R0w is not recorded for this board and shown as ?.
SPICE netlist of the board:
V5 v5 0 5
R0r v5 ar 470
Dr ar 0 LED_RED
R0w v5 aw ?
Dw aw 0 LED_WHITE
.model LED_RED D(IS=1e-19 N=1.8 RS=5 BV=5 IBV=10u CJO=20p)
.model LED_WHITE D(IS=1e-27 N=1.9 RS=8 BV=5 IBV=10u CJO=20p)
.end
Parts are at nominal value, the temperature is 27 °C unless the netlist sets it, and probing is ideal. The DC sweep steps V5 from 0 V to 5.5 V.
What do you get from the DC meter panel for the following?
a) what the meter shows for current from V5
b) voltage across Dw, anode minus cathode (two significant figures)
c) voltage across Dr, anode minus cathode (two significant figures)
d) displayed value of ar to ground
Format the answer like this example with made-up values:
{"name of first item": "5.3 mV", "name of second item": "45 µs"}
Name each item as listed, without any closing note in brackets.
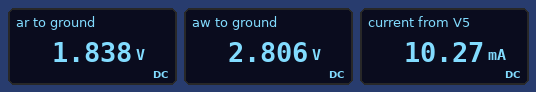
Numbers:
{"what the meter shows for current from V5": "10.27 mA", "voltage across Dw, anode minus cathode": "2.8 V", "voltage across Dr, anode minus cathode": "1.8 V", "displayed value of ar to ground": "1.838 V"}
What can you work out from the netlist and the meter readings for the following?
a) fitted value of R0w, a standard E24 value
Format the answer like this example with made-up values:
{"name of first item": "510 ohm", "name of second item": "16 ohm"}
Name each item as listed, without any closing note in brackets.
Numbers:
{"fitted value of R0w, a standard E24 value": "620 Ω"}
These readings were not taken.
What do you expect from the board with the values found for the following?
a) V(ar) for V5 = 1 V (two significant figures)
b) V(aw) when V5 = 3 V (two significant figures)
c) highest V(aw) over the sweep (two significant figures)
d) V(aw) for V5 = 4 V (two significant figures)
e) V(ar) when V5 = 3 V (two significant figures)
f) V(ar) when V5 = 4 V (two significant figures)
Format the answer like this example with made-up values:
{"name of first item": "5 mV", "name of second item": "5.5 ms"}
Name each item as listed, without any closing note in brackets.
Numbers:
{"V(ar) for V5 = 1 V": "1.0 V", "V(aw) when V5 = 3 V": "2.7 V", "highest V(aw) over the sweep": "2.8 V", "V(aw) for V5 = 4 V": "2.8 V", "V(ar) when V5 = 3 V": "1.8 V", "V(ar) when V5 = 4 V": "1.8 V"}
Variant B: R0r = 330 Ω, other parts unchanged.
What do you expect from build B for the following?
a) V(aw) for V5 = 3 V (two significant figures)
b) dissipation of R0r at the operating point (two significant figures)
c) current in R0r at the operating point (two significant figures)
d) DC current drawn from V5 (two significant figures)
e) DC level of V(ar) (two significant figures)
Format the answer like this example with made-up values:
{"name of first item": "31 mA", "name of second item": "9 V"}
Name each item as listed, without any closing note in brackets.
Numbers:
{"V(aw) for V5 = 3 V": "2.7 V", "dissipation of R0r at the operating point": "30 mW", "current in R0r at the operating point": "9.5 mA", "DC current drawn from V5": "13 mA", "DC level of V(ar)": "1.9 V"}
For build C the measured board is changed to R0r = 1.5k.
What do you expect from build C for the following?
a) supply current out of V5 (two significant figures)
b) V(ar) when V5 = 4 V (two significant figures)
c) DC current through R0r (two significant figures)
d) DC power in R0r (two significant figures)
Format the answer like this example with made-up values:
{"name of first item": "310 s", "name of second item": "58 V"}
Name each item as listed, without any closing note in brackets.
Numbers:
{"supply current out of V5": "5.7 mA", "V(ar) when V5 = 4 V": "1.7 V", "DC current through R0r": "2.2 mA", "DC power in R0r": "7.0 mW"}
